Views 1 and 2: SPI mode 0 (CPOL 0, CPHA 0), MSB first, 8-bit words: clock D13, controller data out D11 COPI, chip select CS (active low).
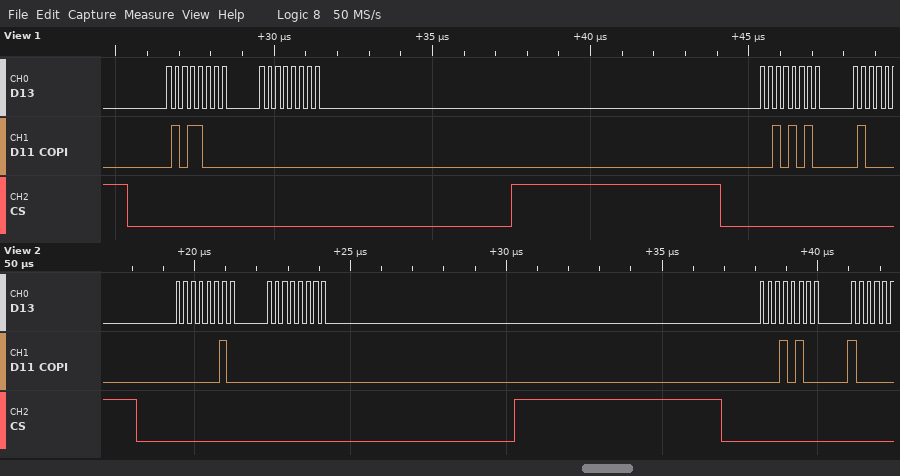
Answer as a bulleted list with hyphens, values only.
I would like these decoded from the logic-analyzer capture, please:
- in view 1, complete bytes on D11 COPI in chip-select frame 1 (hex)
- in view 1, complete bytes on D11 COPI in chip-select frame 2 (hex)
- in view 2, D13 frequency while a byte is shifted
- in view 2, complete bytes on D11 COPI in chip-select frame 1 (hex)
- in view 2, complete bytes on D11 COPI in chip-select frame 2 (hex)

- 58 00
- 2A
- 4 MHz
- 0x02 0x00
- 0x14
